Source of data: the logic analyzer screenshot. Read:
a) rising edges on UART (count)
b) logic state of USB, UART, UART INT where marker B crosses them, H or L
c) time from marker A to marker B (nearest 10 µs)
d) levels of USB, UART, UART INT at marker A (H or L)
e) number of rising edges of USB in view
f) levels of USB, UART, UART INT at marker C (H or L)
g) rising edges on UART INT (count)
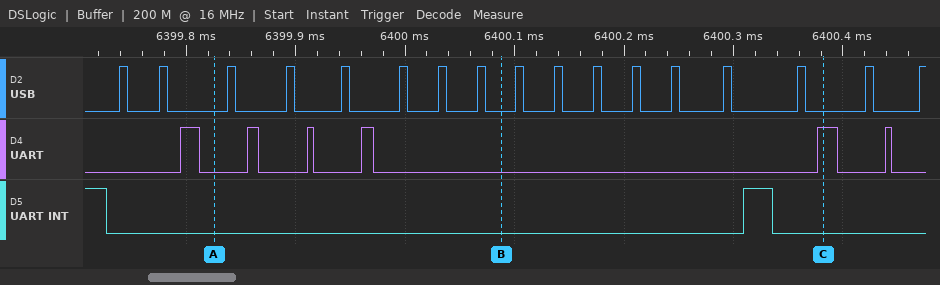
6
USB=L, UART=L, UART INT=L
260 µs
USB=L, UART=L, UART INT=L
17
USB=L, UART=H, UART INT=L
1
